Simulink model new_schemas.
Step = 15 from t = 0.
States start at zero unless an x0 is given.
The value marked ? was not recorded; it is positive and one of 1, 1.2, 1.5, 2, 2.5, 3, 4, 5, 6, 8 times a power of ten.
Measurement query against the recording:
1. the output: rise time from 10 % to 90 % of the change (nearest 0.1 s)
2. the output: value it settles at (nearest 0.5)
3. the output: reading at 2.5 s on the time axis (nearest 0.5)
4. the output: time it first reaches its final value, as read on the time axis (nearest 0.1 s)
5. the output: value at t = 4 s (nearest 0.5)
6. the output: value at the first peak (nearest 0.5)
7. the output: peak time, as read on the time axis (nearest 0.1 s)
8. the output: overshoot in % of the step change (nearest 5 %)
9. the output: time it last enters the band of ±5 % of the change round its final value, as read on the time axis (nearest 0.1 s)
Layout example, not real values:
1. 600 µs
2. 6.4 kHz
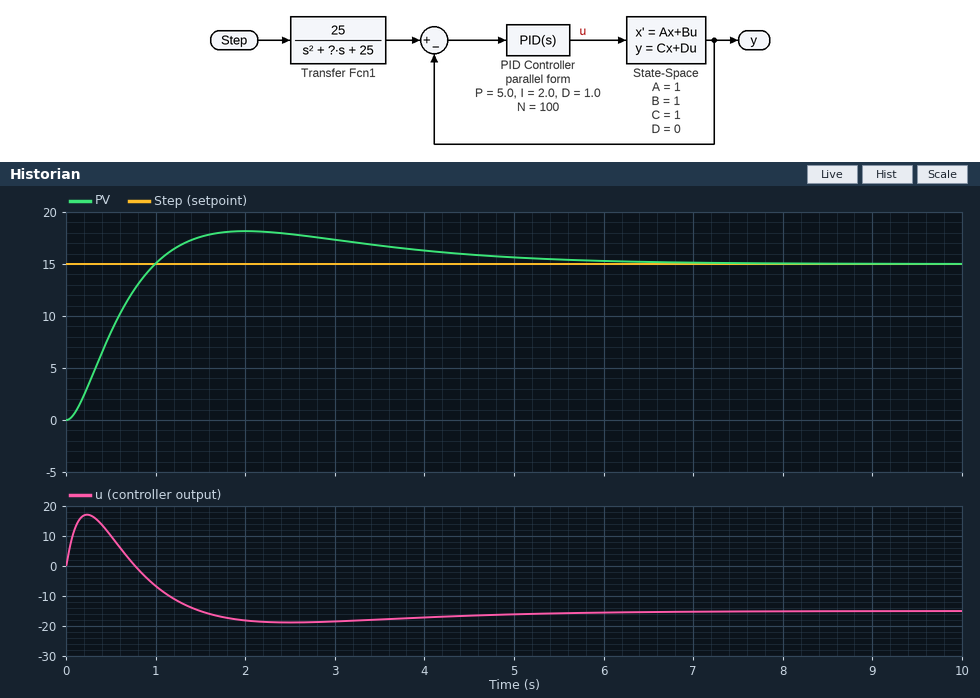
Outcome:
1. 0.7 s
2. 15.0
3. 18.0
4. 1.0 s
5. 16.5
6. 18.0
7. 2.0 s
8. 20 %
9. 4.8 s
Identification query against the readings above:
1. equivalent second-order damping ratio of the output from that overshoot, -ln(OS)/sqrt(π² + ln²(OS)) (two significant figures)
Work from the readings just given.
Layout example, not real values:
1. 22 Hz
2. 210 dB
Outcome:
1. 0.46
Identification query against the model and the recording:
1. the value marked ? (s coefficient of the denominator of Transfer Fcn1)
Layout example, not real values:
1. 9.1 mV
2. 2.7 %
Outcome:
1. 10
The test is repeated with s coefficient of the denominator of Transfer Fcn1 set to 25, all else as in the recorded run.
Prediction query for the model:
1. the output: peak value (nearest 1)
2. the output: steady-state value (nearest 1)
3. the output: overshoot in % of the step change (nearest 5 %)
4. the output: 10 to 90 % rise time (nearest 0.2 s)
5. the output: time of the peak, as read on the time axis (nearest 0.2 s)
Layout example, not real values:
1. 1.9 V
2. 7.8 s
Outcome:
1. 17
2. 15
3. 10 %
4. 1.4 s
5. 3.2 s
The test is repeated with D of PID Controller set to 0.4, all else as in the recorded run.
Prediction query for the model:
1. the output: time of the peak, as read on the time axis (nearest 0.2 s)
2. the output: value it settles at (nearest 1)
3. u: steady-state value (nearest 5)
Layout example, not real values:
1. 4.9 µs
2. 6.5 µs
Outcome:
1. 1.8 s
2. 15
3. -15
